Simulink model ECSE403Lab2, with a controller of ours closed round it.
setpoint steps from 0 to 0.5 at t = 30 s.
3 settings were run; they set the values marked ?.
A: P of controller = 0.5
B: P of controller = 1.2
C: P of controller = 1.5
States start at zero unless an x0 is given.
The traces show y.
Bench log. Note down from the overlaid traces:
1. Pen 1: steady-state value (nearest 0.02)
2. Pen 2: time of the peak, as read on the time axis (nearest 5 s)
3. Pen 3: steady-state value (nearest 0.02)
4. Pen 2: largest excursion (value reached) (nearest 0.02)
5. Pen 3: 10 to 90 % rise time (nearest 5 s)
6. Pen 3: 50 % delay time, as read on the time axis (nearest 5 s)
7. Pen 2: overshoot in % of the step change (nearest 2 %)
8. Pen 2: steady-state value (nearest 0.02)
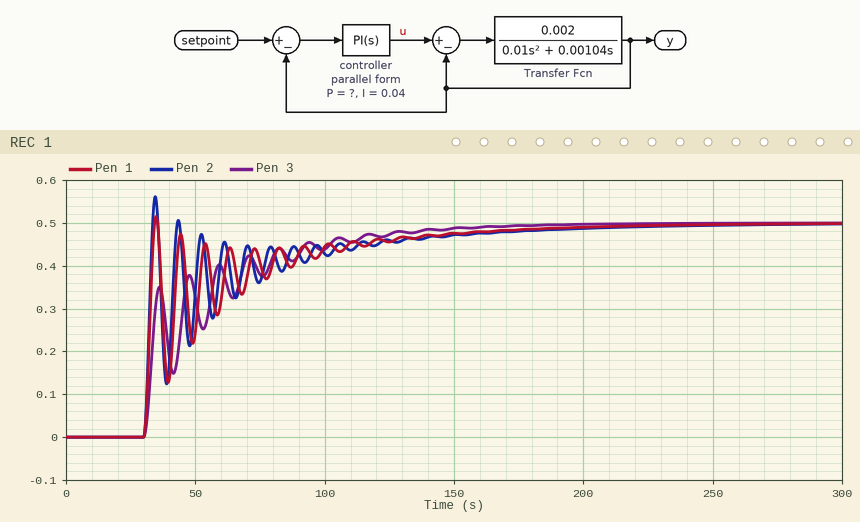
0.50
35 s
0.50
0.56
60 s
35 s
12 %
0.50
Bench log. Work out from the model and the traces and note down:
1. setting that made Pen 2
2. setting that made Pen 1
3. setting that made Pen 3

C
B
A
